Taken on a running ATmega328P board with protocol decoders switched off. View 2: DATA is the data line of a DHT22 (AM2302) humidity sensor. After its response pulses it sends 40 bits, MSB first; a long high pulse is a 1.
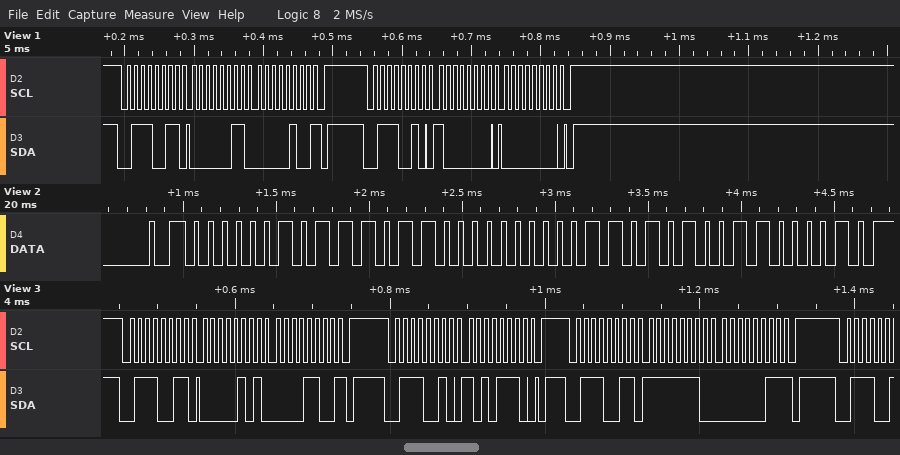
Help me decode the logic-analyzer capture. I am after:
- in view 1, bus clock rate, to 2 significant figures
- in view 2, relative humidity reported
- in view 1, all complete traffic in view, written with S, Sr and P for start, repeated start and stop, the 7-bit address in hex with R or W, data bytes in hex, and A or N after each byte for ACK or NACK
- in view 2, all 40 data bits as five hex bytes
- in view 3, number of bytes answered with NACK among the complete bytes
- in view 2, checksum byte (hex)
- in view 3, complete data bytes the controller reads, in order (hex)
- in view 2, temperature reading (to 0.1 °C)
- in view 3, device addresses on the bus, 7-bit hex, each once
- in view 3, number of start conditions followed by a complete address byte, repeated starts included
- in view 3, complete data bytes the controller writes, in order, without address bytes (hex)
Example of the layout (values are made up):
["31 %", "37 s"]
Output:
["100 kHz", "74.8 %", "S 39R A 03 A 04 N P S 39W A 80 A 00 A P", "02 EC 00 D4 C2", "2", "0xC2", "05 0C FE 03", "21.2 °C", "0x39", "3", "AE"]
